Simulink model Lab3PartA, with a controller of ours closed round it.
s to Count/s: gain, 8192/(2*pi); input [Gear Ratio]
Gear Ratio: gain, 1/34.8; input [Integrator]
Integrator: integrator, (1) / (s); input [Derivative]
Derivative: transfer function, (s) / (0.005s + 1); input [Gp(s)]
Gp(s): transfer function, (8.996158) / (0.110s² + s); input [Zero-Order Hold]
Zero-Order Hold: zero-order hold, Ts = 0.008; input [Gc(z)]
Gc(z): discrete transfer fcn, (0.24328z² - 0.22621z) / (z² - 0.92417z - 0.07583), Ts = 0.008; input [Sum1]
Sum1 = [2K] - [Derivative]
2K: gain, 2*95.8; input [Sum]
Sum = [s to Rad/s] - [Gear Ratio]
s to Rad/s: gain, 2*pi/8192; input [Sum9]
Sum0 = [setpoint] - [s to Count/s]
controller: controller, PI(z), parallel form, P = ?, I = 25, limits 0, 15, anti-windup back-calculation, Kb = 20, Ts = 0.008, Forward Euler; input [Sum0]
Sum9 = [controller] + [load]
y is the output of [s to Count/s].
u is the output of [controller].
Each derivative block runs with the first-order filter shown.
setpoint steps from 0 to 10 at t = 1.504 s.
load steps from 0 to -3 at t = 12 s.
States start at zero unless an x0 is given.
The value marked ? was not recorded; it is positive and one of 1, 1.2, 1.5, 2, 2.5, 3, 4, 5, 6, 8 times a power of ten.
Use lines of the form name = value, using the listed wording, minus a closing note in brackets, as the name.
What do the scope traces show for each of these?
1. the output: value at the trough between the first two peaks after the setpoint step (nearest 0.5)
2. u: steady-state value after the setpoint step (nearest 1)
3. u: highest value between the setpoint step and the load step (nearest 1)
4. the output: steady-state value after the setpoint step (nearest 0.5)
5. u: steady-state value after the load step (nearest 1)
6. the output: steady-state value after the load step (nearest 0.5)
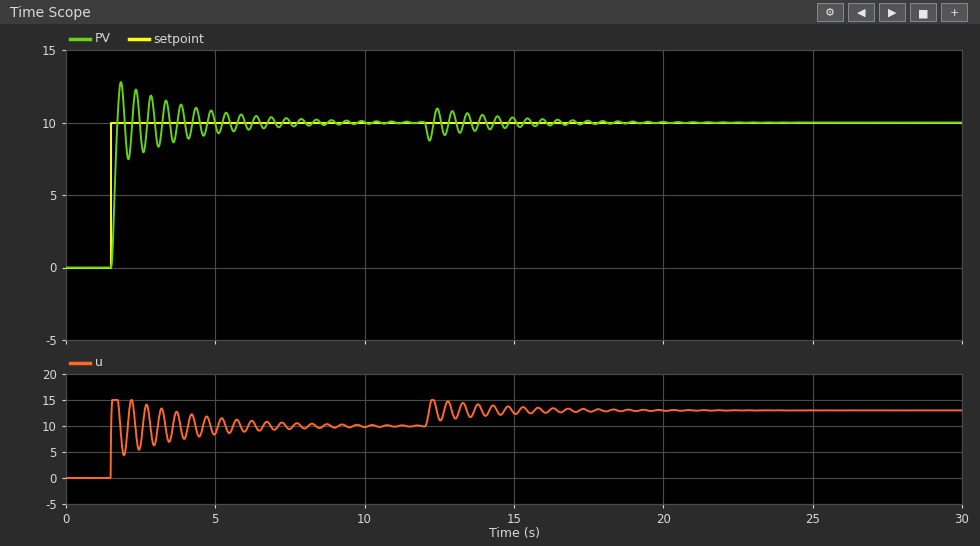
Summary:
the output: value at the trough between the first two peaks after the setpoint step = 7.5
u: steady-state value after the setpoint step = 10
u: highest value between the setpoint step and the load step = 15
the output: steady-state value after the setpoint step = 10.0
u: steady-state value after the load step = 13
the output: steady-state value after the load step = 10.0
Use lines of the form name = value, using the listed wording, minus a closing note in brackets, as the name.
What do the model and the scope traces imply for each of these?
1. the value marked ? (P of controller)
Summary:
the value marked ? = 0.8
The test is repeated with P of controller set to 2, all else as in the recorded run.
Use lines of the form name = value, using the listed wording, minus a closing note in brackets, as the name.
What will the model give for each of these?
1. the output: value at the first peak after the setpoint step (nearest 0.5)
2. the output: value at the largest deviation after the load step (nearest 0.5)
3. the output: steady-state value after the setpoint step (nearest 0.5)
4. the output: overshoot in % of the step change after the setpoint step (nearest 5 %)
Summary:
the output: value at the first peak after the setpoint step = 11.5
the output: value at the largest deviation after the load step = 9.0
the output: steady-state value after the setpoint step = 10.0
the output: overshoot in % of the step change after the setpoint step = 15 %
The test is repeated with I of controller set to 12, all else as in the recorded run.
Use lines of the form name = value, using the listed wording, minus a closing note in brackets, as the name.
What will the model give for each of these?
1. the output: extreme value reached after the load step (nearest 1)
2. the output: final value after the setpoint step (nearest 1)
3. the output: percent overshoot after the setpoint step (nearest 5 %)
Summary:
the output: extreme value reached after the load step = 9
the output: final value after the setpoint step = 10
the output: percent overshoot after the setpoint step = 25 %
